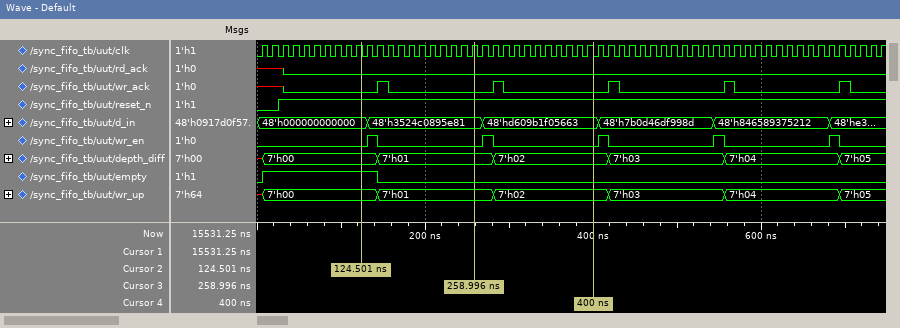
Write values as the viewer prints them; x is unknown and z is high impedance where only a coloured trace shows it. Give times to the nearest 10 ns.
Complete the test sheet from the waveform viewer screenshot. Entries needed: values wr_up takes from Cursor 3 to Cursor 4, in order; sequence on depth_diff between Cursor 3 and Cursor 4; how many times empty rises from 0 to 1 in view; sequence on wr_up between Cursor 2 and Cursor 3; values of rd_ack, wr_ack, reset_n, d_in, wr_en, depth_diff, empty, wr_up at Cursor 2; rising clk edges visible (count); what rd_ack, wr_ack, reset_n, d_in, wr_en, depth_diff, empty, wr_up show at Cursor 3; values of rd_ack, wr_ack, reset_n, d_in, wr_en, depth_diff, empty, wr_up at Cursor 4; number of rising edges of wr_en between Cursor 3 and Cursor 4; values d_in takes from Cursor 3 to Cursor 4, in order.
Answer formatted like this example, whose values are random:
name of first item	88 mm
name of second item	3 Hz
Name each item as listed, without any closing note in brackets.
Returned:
values wr_up takes from Cursor 3 to Cursor 4, in order	7'h01, 7'h02
sequence on depth_diff between Cursor 3 and Cursor 4	7'h01, 7'h02
how many times empty rises from 0 to 1 in view	1
sequence on wr_up between Cursor 2 and Cursor 3	7'h00, 7'h01
values of rd_ack, wr_ack, reset_n, d_in, wr_en, depth_diff, empty, wr_up at Cursor 2	rd_ack=0, wr_ack=0, reset_n=1, d_in=48'h000000000000, wr_en=0, depth_diff=7'h00, empty=1, wr_up=7'h00
rising clk edges visible	60
what rd_ack, wr_ack, reset_n, d_in, wr_en, depth_diff, empty, wr_up show at Cursor 3	rd_ack=0, wr_ack=0, reset_n=1, d_in=48'h3524c0895e81, wr_en=0, depth_diff=7'h01, empty=0, wr_up=7'h01
values of rd_ack, wr_ack, reset_n, d_in, wr_en, depth_diff, empty, wr_up at Cursor 4	rd_ack=0, wr_ack=0, reset_n=1, d_in=48'hd609b1f05663, wr_en=0, depth_diff=7'h02, empty=0, wr_up=7'h02
number of rising edges of wr_en between Cursor 3 and Cursor 4	1
values d_in takes from Cursor 3 to Cursor 4, in order	48'h3524c0895e81, 48'hd609b1f05663
